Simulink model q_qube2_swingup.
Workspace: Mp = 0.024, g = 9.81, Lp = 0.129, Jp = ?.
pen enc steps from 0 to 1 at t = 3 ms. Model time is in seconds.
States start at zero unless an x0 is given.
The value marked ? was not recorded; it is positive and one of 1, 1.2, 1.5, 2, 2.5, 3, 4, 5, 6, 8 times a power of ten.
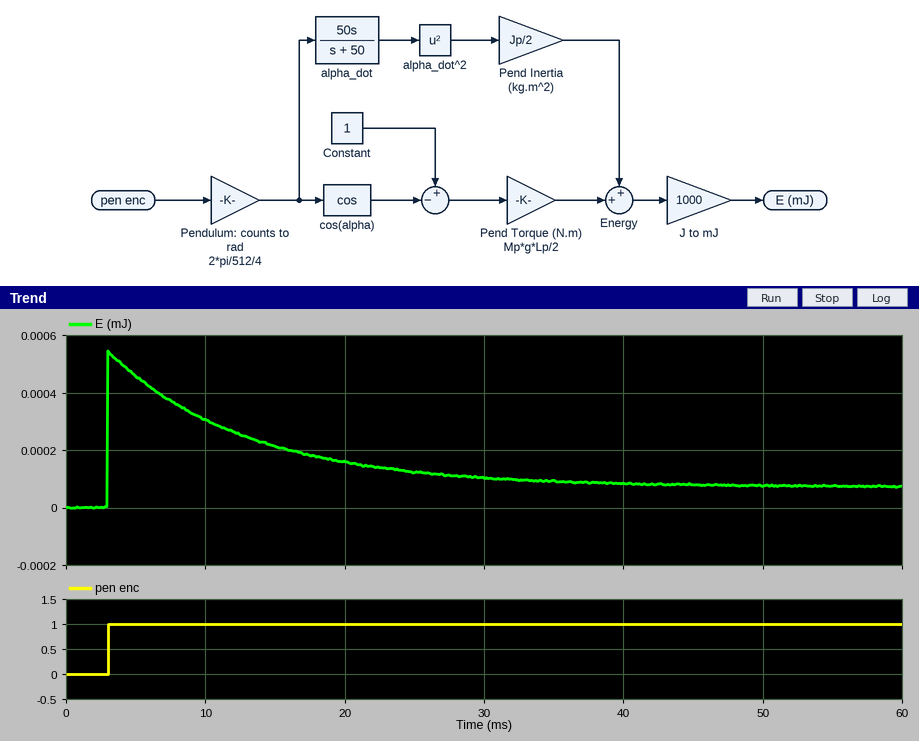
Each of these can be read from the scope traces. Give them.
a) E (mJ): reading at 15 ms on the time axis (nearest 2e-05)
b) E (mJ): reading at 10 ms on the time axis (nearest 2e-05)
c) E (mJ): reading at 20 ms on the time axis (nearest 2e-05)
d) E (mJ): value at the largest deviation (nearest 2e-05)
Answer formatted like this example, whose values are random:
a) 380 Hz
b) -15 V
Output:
a) 0.00022
b) 0.00030
c) 0.00016
d) 0.00054
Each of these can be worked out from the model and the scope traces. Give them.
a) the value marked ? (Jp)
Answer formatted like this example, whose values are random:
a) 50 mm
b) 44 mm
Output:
a) 4e-05
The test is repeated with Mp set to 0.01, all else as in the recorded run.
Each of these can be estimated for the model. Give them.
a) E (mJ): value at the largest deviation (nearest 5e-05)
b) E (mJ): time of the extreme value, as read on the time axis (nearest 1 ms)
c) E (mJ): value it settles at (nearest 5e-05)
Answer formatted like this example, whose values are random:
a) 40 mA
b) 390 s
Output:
a) 0.00050
b) 3 ms
c) 0.00005
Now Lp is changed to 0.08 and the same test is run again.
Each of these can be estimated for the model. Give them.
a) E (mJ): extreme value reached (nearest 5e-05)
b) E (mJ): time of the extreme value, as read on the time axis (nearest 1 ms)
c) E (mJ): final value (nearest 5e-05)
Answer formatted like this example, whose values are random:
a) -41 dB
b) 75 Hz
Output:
a) 0.00050
b) 3 ms
c) 0.00005
